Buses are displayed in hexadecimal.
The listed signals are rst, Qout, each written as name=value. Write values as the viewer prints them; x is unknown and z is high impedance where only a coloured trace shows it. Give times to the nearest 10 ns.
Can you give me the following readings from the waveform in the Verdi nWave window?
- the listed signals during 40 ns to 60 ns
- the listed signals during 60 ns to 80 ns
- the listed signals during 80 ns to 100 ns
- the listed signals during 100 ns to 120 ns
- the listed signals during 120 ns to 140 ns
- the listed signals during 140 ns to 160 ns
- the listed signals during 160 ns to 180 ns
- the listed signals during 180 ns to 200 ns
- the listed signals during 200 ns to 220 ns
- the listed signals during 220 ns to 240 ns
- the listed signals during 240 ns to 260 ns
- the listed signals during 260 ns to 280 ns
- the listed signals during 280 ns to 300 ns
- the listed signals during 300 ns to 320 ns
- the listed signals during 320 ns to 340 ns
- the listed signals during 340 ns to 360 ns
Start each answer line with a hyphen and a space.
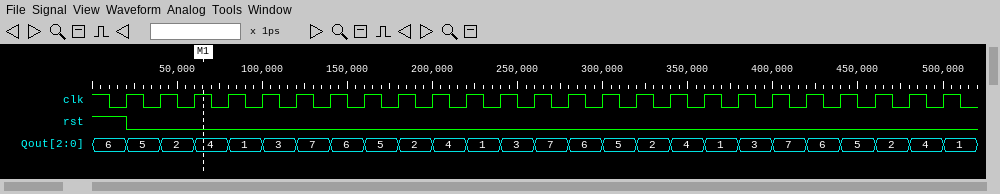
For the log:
- rst=0, Qout=2
- rst=0, Qout=4
- rst=0, Qout=1
- rst=0, Qout=3
- rst=0, Qout=7
- rst=0, Qout=6
- rst=0, Qout=5
- rst=0, Qout=2
- rst=0, Qout=4
- rst=0, Qout=1
- rst=0, Qout=3
- rst=0, Qout=7
- rst=0, Qout=6
- rst=0, Qout=5
- rst=0, Qout=2
- rst=0, Qout=4
